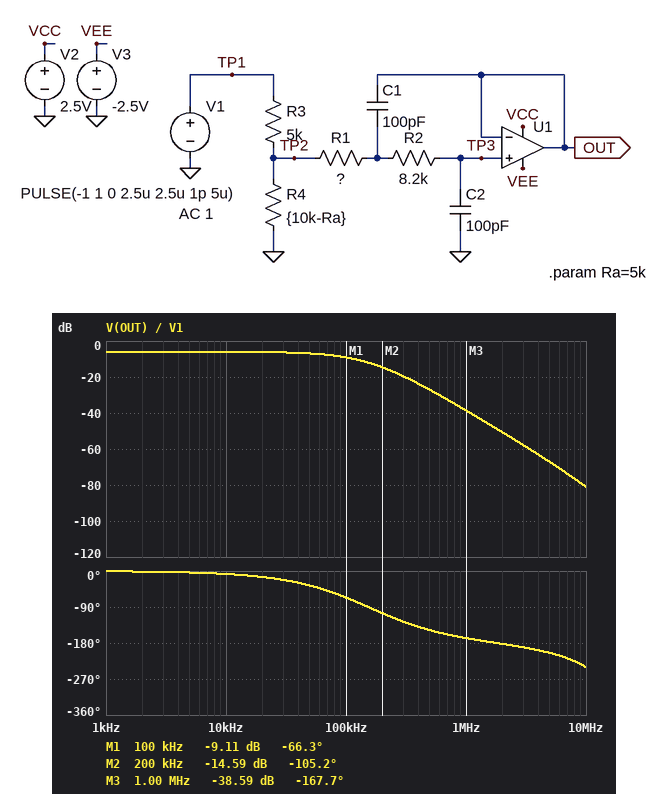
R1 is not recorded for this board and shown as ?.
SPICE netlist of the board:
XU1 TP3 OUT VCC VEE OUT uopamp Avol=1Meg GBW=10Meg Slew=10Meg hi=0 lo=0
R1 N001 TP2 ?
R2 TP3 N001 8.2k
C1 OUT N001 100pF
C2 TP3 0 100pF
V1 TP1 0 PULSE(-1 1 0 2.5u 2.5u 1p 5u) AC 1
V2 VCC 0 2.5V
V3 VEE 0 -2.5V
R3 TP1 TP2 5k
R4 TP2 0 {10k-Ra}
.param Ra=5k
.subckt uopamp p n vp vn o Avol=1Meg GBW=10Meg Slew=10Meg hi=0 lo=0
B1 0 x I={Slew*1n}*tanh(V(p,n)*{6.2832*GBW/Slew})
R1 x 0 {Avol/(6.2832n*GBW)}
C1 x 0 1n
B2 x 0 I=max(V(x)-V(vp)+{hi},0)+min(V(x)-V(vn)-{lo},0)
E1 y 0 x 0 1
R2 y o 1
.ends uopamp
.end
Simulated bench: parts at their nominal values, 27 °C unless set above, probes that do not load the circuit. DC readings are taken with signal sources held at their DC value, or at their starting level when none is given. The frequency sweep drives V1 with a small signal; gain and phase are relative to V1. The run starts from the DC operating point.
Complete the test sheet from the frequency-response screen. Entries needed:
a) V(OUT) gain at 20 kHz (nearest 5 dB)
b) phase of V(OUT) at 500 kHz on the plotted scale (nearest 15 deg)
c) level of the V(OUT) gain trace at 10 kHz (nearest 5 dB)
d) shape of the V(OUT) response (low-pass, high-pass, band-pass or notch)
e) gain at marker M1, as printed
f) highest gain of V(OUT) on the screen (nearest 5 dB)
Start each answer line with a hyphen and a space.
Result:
- -5 dB
- -150 deg
- -5 dB
- low-pass
- -9.11 dB
- -5 dB
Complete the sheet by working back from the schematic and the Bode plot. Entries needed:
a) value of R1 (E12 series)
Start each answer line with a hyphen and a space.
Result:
- 10 kΩ
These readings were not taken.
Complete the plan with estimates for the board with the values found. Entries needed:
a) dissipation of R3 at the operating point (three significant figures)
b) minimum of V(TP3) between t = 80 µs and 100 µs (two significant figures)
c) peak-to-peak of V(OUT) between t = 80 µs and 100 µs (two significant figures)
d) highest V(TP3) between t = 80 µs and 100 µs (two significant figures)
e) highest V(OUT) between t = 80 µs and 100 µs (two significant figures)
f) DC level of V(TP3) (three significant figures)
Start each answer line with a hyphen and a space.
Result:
- 50.0 µW
- -150 mV
- 300 mV
- 150 mV
- 150 mV
- -500 mV
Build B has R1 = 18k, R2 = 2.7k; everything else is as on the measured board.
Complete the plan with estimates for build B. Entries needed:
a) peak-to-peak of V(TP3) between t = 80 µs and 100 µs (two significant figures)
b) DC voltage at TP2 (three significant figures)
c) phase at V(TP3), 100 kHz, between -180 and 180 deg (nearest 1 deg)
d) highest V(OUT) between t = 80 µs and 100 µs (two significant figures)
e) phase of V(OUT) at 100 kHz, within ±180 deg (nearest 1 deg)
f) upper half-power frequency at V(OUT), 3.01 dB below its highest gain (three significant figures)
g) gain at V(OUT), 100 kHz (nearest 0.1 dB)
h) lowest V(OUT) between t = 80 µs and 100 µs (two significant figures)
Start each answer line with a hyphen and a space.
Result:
- 270 mV
- -500 mV
- -62 deg
- 140 mV
- -63 deg
- 76.8 kHz
- -10.4 dB
- -140 mV
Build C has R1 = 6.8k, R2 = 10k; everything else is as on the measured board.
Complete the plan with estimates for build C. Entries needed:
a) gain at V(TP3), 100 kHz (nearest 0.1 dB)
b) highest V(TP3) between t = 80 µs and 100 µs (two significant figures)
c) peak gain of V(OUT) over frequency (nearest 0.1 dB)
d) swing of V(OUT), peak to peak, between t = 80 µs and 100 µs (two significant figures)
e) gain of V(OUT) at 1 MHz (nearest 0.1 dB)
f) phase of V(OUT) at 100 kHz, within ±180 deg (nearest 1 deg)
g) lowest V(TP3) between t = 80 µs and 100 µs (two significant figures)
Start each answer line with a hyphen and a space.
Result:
- -8.7 dB
- 160 mV
- -6.0 dB
- 320 mV
- -37.7 dB
- -63 deg
- -160 mV
